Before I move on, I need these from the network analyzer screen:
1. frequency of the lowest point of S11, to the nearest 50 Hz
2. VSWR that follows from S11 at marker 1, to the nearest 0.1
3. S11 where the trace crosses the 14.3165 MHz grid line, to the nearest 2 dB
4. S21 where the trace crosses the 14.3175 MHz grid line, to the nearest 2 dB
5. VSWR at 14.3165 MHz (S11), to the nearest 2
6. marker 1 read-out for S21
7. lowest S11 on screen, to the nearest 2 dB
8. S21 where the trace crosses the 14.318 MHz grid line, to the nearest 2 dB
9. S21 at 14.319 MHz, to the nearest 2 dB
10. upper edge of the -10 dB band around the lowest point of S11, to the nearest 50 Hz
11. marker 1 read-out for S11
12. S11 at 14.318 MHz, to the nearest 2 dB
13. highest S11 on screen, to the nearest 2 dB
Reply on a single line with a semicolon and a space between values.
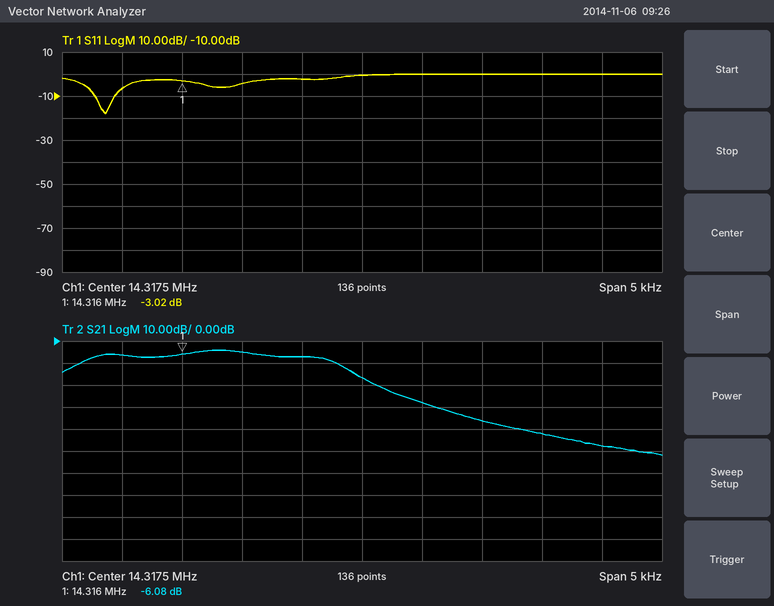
14.31535 MHz; 5.8; -4 dB; -16 dB; 4; -6.08 dB; -18 dB; -28 dB; -42 dB; 14.31545 MHz; -3.02 dB; 0 dB; 0 dB
